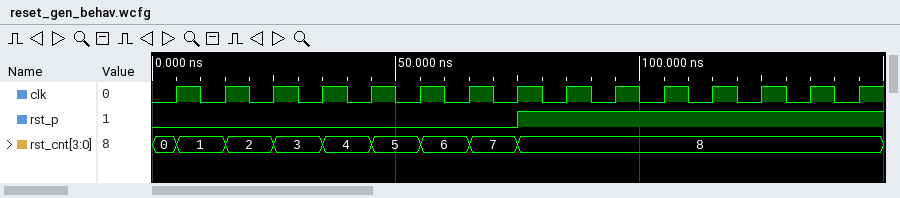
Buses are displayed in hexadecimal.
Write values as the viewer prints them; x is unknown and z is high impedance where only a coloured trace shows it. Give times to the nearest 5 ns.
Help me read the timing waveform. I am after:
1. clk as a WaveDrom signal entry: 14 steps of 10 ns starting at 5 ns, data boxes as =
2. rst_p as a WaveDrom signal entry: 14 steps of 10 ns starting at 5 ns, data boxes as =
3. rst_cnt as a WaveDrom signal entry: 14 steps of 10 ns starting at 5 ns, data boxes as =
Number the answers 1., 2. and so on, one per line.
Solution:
1. {name: 'clk', wave: 'p.............'}
2. {name: 'rst_p', wave: '0......1......'}
3. {name: 'rst_cnt', wave: '========......', data: '1 2 3 4 5 6 7 8'}
